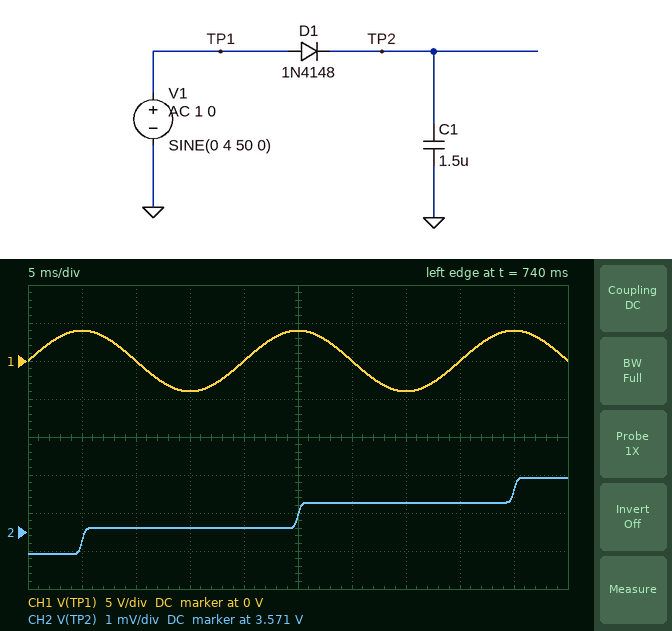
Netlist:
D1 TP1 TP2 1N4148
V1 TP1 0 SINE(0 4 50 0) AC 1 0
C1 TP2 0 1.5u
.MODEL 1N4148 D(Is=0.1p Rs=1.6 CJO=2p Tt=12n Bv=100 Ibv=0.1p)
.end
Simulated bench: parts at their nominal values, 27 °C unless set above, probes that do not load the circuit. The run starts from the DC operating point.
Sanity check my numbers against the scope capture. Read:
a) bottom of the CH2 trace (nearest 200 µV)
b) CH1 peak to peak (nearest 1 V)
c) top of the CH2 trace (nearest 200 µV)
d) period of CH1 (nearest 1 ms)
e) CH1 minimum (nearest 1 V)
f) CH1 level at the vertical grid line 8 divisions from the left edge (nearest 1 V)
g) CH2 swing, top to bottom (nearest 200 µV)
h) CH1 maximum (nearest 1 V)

3.5704 V
8 V
3.5724 V
20 ms
-4 V
0 V
2.0 mV
4 V
